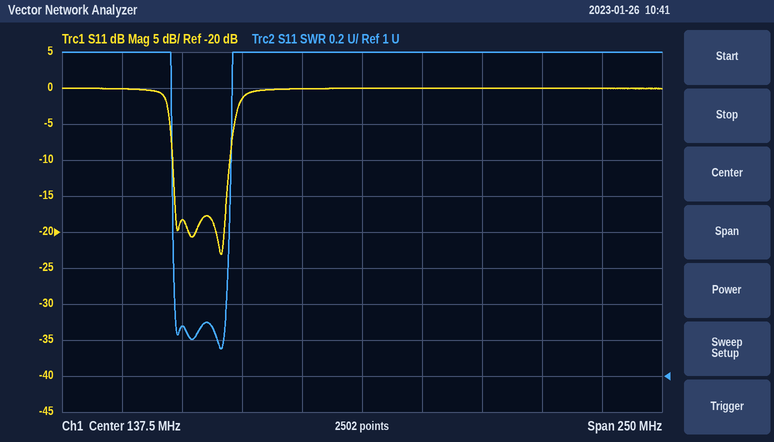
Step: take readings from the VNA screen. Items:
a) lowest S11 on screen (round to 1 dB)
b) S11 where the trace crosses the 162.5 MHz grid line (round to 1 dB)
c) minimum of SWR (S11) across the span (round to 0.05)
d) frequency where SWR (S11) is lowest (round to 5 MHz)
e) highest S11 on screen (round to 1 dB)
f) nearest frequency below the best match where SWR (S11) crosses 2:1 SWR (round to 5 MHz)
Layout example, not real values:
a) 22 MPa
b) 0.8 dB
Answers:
a) -23 dB
b) 0 dB
c) 1.15
d) 80 MHz
e) 0 dB
f) 60 MHz
